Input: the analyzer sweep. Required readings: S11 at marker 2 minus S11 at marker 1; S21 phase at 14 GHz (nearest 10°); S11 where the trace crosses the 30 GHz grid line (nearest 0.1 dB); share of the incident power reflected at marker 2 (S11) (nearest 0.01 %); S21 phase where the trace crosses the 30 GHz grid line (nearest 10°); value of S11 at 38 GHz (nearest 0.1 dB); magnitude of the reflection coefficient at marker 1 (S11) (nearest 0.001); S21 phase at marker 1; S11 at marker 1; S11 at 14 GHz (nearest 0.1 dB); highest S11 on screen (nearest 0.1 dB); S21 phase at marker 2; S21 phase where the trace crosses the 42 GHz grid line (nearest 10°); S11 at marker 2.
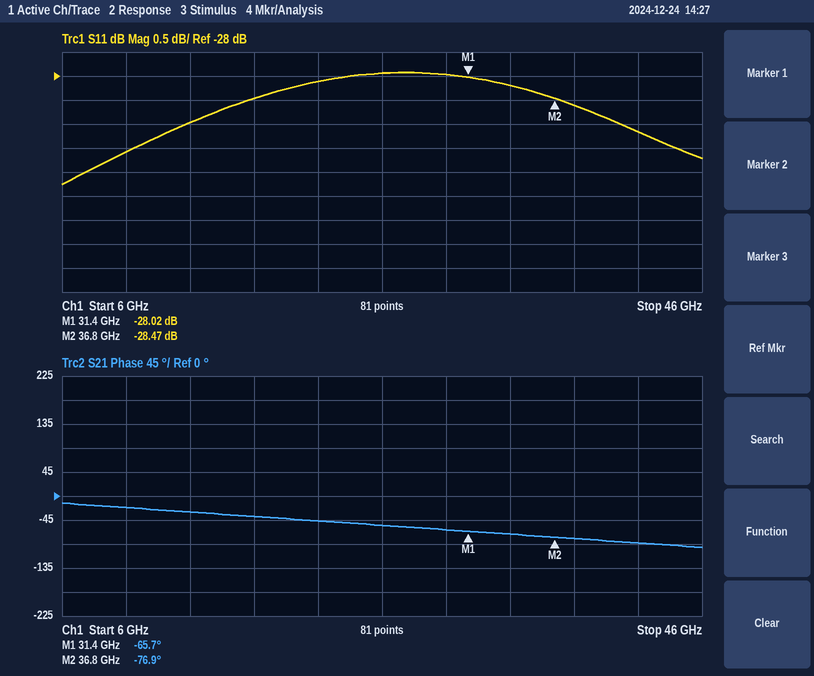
-0.45 dB
-30°
-28.0 dB
0.14 %
-60°
-28.6 dB
0.040
-65.7°
-28.02 dB
-29.0 dB
-27.9 dB
-76.9°
-90°
-28.47 dB
